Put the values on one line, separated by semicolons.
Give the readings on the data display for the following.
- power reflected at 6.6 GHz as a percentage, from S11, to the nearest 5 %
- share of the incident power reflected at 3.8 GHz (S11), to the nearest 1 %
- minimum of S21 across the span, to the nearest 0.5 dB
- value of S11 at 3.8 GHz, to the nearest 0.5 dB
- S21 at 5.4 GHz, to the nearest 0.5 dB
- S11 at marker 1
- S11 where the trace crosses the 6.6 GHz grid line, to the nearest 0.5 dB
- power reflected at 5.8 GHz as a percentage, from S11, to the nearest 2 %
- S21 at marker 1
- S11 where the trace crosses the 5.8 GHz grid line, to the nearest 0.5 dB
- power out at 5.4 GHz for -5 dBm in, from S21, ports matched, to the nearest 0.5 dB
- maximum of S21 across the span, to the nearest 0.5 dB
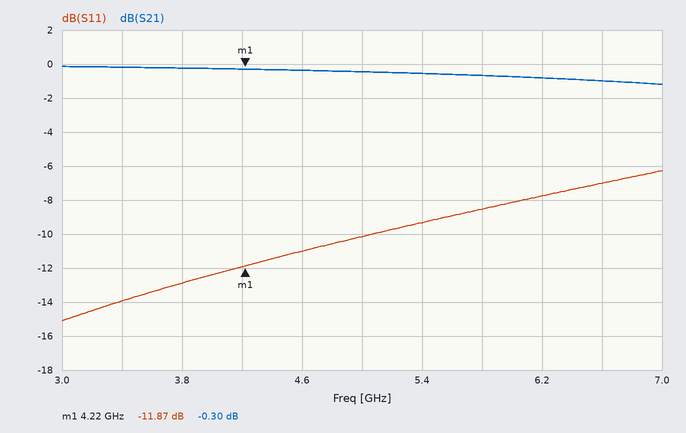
20 %; 5 %; -1.0 dB; -13.0 dB; -0.5 dB; -11.87 dB; -7.0 dB; 14 %; -0.30 dB; -8.5 dB; -5.5 dBm; 0.0 dB
